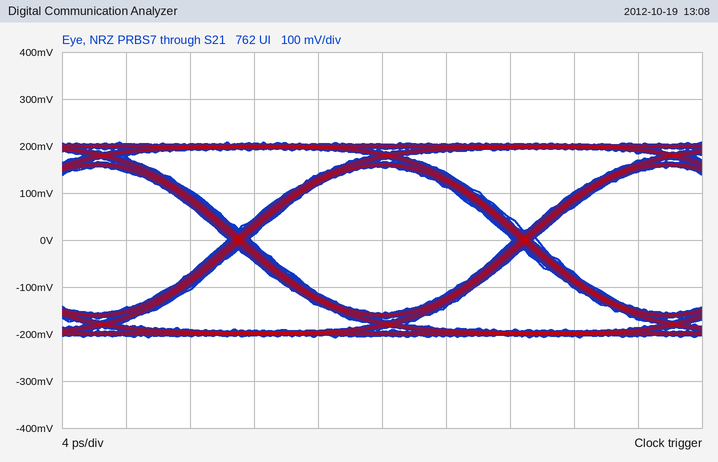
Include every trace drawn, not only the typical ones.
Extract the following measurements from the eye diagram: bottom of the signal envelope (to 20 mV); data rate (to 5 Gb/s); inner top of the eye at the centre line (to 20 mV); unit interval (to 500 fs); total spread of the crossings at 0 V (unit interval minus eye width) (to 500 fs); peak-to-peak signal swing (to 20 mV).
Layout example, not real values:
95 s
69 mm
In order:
-200 mV
55 Gb/s
160 mV
18.0 ps
1.5 ps
420 mV
